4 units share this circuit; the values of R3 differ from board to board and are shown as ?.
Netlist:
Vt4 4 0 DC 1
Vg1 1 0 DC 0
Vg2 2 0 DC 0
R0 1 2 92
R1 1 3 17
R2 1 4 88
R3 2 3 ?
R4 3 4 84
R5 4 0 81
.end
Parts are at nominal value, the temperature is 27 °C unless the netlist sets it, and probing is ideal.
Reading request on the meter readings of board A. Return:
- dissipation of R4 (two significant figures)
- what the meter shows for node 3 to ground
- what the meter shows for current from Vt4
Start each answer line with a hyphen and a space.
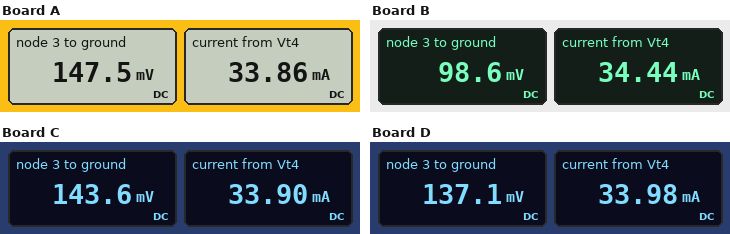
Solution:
- 8.7 mW
- 147.5 mV
- 33.86 mA
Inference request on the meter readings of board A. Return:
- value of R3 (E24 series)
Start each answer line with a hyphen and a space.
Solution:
- 100 Ω
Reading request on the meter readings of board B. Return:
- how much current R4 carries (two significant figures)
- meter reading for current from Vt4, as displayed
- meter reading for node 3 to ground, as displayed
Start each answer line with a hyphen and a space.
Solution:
- 11 mA
- 34.44 mA
- 98.6 mV
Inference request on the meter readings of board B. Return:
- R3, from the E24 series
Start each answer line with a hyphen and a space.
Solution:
- 20 Ω
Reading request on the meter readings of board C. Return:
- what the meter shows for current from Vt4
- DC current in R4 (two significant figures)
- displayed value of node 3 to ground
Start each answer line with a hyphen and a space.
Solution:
- 33.90 mA
- 10 mA
- 143.6 mV
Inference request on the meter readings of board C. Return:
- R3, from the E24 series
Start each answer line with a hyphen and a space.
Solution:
- 82 Ω
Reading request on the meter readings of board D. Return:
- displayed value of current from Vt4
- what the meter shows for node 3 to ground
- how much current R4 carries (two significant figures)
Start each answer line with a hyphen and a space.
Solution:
- 33.98 mA
- 137.1 mV
- 10 mA
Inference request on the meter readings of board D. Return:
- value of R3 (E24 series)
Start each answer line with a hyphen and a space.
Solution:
- 62 Ω
